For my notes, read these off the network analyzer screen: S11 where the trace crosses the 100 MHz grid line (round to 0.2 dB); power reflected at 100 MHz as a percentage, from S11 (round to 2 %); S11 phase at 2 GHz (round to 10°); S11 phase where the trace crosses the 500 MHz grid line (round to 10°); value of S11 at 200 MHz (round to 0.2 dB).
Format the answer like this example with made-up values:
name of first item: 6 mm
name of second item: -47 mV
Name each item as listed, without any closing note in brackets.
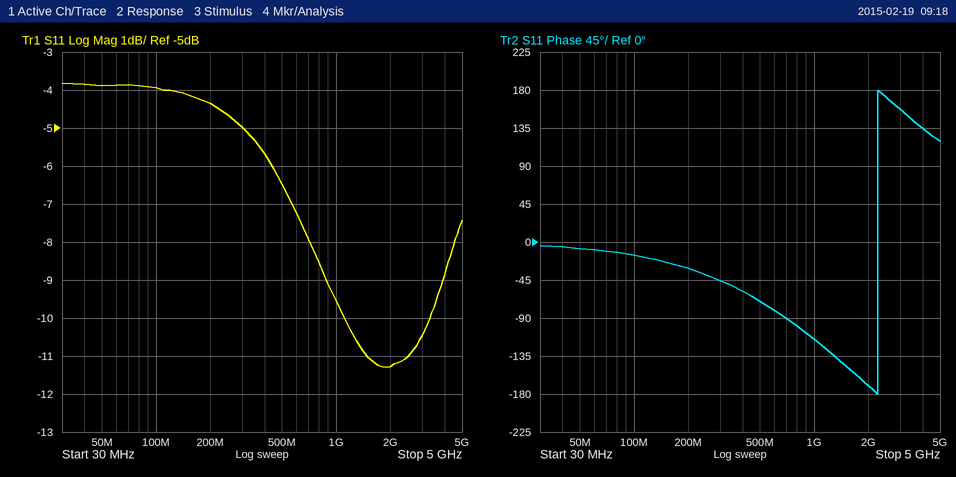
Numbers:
S11 where the trace crosses the 100 MHz grid line: -4.0 dB
power reflected at 100 MHz as a percentage, from S11: 40 %
S11 phase at 2 GHz: -170°
S11 phase where the trace crosses the 500 MHz grid line: -70°
value of S11 at 200 MHz: -4.4 dB
